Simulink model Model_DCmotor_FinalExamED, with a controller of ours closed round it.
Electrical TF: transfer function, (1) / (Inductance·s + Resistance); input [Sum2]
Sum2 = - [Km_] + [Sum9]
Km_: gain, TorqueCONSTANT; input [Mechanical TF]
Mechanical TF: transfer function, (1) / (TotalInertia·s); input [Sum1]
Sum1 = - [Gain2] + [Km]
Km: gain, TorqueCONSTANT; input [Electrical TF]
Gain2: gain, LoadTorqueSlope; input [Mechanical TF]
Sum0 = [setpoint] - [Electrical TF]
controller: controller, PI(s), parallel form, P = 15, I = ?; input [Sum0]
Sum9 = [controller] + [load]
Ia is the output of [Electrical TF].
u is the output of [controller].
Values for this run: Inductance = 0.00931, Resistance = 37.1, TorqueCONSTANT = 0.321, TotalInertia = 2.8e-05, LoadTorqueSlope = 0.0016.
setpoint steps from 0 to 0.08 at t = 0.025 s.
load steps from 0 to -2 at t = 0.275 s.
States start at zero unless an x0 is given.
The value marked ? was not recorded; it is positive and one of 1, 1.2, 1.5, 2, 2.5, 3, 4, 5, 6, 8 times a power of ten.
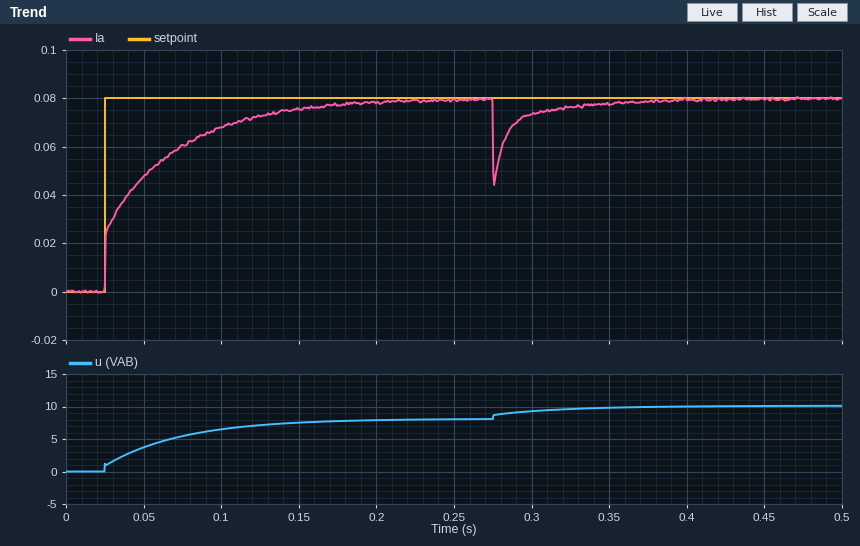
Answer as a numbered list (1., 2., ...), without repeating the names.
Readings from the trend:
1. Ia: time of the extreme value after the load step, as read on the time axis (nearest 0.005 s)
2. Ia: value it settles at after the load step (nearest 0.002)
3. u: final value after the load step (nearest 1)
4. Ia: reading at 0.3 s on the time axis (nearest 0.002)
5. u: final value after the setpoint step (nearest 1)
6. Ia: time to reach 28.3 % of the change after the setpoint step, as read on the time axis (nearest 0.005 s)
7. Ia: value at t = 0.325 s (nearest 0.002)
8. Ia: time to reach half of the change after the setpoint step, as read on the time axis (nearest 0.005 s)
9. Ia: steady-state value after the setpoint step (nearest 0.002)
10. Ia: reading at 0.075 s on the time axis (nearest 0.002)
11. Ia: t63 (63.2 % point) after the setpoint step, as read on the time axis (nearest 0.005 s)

1. 0.275 s
2. 0.080
3. 10
4. 0.074
5. 8
6. 0.025 s
7. 0.076
8. 0.040 s
9. 0.080
10. 0.060
11. 0.055 s
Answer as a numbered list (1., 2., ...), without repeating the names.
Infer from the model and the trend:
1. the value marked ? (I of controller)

1. 3000
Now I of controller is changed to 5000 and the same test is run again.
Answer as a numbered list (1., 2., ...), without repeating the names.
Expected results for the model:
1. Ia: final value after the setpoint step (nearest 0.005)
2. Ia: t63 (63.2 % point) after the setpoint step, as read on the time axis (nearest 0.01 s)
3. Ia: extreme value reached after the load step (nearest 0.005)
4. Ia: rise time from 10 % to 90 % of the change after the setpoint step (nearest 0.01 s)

1. 0.080
2. 0.04 s
3. 0.045
4. 0.06 s
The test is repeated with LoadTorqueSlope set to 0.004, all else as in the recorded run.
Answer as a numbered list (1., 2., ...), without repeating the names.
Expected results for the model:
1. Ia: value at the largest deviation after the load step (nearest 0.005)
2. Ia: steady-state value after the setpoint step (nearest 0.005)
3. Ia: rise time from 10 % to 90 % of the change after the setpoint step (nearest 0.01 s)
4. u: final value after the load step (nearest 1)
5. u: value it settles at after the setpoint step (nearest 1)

1. 0.045
2. 0.080
3. 0.06 s
4. 7
5. 5
